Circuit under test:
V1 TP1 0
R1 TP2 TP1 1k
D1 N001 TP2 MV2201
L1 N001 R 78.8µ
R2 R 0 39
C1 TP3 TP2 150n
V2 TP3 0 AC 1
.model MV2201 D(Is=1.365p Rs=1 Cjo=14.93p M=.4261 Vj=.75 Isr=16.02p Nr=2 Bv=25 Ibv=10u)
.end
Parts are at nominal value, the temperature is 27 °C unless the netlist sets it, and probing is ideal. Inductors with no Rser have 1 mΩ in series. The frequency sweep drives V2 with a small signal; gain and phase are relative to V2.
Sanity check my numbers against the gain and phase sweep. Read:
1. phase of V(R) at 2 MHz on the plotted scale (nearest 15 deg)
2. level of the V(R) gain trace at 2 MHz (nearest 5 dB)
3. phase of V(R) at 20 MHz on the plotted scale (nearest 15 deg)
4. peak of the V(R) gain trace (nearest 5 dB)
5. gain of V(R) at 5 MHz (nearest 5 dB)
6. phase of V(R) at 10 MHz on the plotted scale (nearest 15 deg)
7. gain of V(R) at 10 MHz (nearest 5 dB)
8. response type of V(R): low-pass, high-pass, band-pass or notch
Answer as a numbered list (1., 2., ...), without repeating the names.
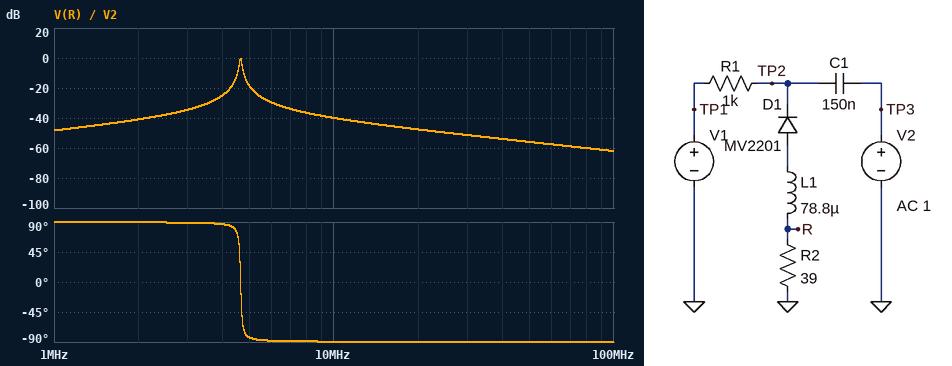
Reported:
1. 90 deg
2. -40 dB
3. -90 deg
4. 0 dB
5. -20 dB
6. -90 deg
7. -40 dB
8. band-pass
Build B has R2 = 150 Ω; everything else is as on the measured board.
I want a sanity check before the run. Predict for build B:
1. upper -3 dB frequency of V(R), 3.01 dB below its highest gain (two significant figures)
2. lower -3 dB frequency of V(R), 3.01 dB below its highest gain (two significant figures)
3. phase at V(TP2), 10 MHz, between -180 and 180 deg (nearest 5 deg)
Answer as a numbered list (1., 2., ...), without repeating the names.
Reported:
1. 4.8 MHz
2. 4.5 MHz
3. 0 deg
